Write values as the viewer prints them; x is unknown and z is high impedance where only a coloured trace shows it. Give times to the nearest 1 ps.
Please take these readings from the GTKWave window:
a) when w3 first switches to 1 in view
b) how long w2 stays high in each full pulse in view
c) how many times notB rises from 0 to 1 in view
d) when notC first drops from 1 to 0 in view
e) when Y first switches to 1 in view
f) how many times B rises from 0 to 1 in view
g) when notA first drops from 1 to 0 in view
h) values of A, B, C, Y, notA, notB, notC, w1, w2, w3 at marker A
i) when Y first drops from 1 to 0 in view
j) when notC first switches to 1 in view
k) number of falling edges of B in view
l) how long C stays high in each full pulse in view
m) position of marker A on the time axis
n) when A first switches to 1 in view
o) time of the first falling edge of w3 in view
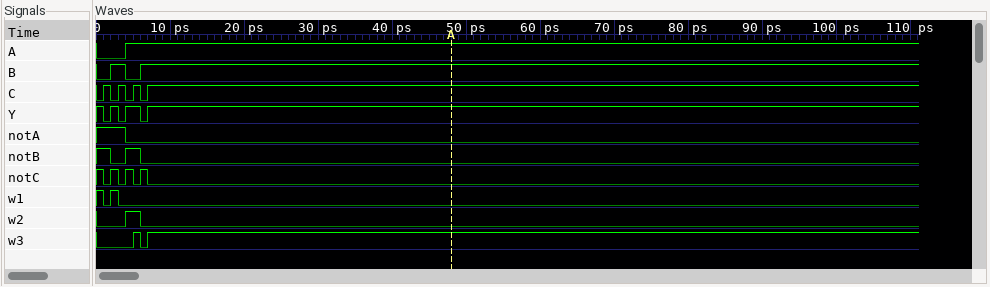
5 ps
2 ps
1
1 ps
2 ps
2
4 ps
A=1, B=1, C=1, Y=1, notA=0, notB=0, notC=0, w1=0, w2=0, w3=1
1 ps
2 ps
1
1 ps, 1 ps, 1 ps
48 ps
4 ps
6 ps
